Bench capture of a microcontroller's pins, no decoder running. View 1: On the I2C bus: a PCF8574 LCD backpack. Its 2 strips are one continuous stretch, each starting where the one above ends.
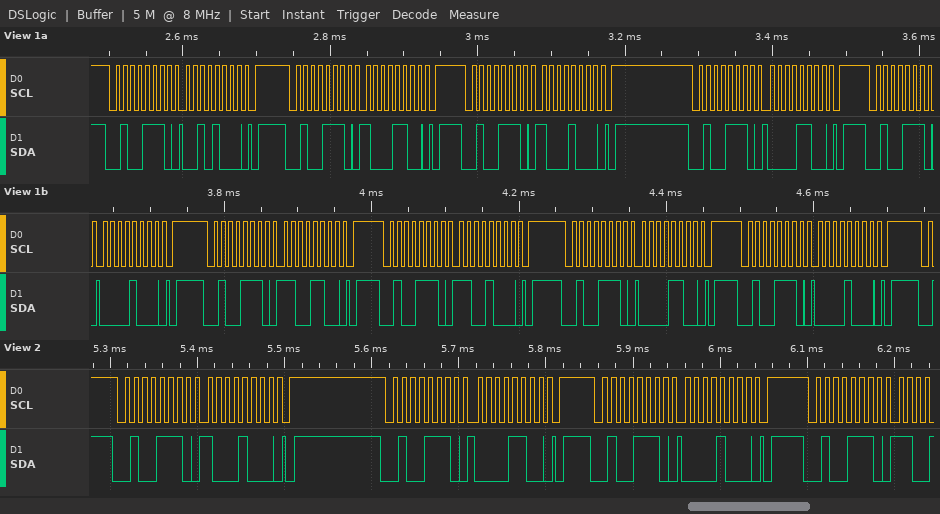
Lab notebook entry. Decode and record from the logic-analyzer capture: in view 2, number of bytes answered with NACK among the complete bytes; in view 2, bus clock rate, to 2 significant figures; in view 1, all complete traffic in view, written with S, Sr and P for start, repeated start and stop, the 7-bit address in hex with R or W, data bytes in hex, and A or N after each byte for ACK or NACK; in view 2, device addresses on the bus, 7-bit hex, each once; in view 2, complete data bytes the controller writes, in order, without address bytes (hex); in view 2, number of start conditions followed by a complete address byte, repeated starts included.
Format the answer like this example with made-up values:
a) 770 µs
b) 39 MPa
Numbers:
a) 0
b) 100 kHz
c) S 27W A 28 A P S 27W A 8C A P S 27W A 88 A P S 27W A 0C A P S 27W A 08 A P S 27W A CC A P S 27W A C8 A P S 27W A 0C A P S 27W A 08 A P
d) 0x27
e) 88 0C 08
f) 4
